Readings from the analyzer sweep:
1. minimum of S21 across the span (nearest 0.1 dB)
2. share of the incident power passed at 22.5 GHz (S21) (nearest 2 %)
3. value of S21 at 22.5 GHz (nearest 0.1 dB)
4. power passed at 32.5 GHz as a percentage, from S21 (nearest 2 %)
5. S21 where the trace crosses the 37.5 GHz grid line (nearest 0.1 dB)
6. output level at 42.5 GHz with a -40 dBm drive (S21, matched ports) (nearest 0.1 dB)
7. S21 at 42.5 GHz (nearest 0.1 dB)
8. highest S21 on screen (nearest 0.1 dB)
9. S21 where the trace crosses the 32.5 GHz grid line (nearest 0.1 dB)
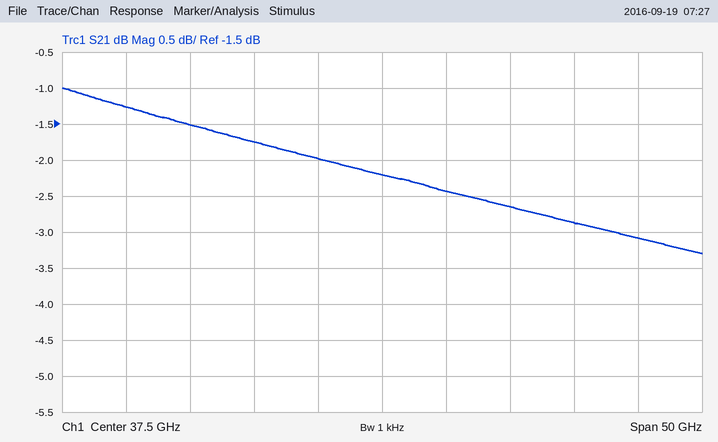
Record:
-3.3 dB
70 %
-1.5 dB
64 %
-2.2 dB
-42.4 dBm
-2.4 dB
-1.0 dB
-2.0 dB
